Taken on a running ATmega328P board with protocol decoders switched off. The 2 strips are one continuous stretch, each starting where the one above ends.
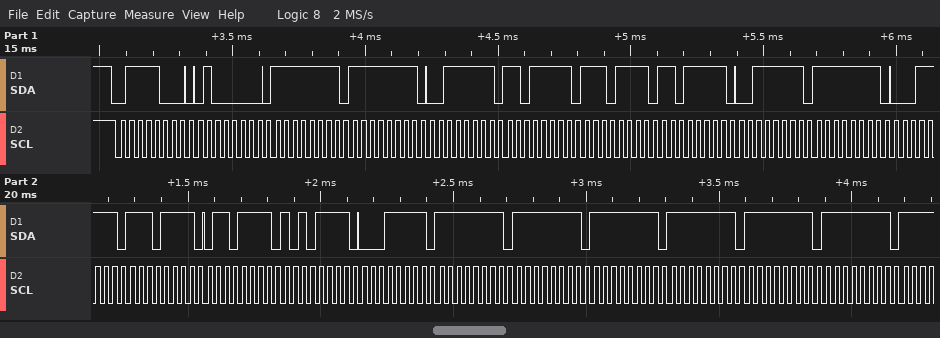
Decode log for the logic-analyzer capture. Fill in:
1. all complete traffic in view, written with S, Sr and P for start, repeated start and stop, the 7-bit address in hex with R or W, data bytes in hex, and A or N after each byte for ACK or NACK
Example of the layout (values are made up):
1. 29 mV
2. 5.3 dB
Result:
1. S 3CW A 40 A FF A FF A 3F A DF A EF A DF A 3F A FF A 1F A EF A 6F A AF A 1F A FF A FF A FF A FF A FF A FF A
